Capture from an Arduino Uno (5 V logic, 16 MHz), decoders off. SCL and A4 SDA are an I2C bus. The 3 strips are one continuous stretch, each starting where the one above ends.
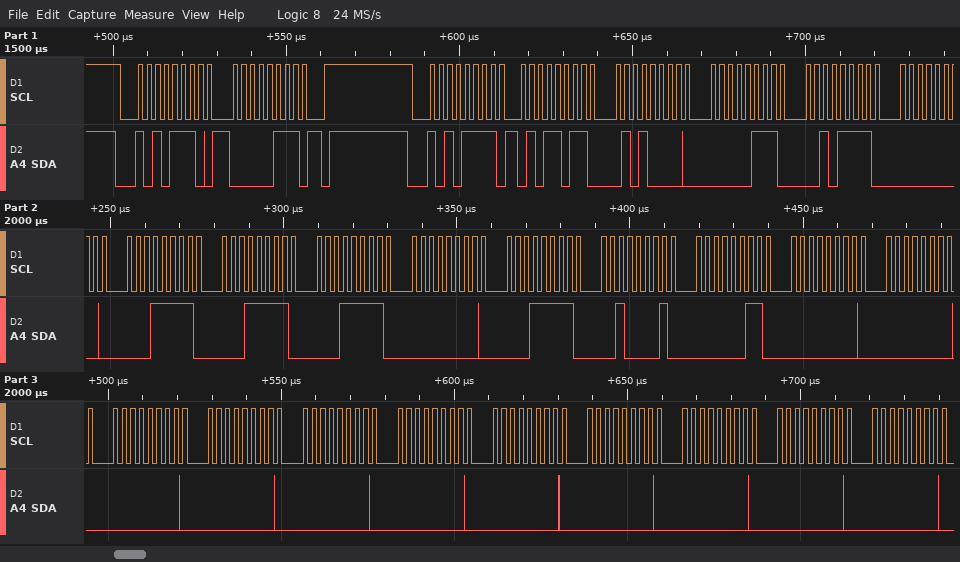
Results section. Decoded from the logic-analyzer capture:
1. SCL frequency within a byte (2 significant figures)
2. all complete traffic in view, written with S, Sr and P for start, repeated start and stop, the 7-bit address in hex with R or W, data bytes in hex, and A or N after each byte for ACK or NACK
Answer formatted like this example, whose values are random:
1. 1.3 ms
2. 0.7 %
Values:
1. 400 kHz
2. S 57W A 07 A P S 57R A 5B A 50 A 07 A 2F A 00 A 1F A 1F A 1F A 00 A 1F A 21 A 03 A 00 A 00 A 00 A 00 A 00 A 00 A 00 A 00 A 00 A 00 A 00 A
